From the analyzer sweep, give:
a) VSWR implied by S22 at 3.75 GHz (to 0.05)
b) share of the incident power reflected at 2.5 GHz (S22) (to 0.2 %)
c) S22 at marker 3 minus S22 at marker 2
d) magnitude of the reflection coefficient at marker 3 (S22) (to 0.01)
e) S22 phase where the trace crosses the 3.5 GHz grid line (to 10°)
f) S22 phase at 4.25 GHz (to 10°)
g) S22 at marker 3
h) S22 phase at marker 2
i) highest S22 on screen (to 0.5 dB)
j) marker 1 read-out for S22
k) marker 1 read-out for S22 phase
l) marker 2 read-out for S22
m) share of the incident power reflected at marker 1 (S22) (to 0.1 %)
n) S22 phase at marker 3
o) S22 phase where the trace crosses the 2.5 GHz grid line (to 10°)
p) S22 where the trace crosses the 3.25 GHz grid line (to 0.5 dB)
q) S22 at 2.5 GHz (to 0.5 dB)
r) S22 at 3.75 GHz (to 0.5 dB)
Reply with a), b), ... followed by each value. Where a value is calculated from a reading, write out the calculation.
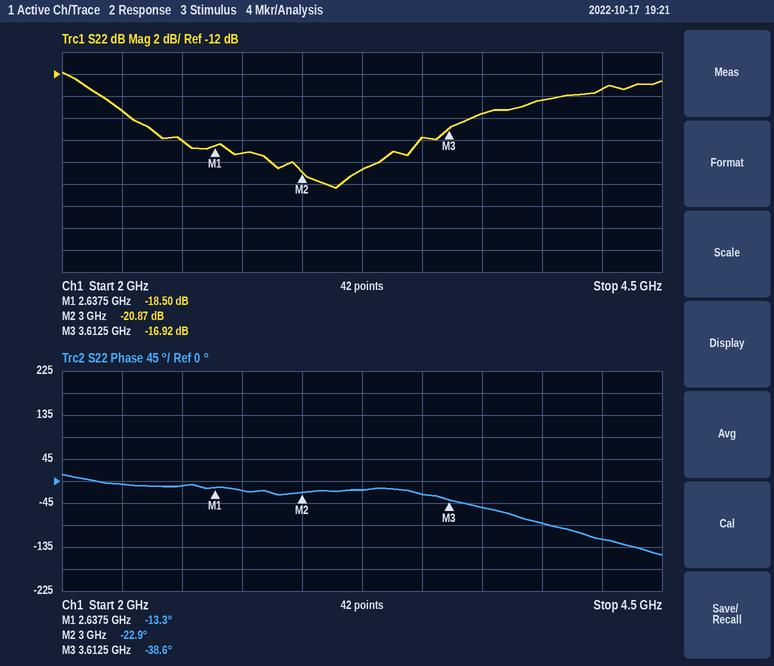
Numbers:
a) |Γ| = 10^(-15.5/20) = 0.1679; VSWR = (1 + 0.1679)/(1 − 0.1679) ≈ 1.40
b) 10^(-18/10) ≈ 1.6 %
c) -16.92 − (-20.87) = 3.95 dB
d) 10^(-16.92/20) ≈ 0.14
e) -30°
f) -120°
g) -16.92 dB
h) -22.9°
i) -12.0 dB
j) -18.50 dB
k) -13.3°
l) -20.87 dB
m) 10^(-18.5/10) ≈ 1.4 %
n) -38.6°
o) -10°
p) -20.5 dB
q) -18.0 dB
r) -15.5 dB
